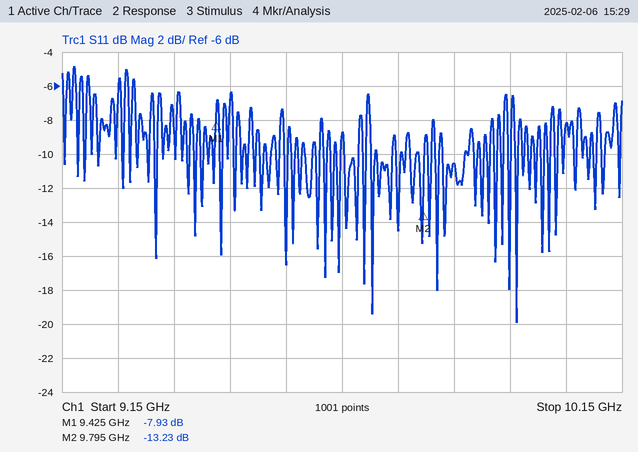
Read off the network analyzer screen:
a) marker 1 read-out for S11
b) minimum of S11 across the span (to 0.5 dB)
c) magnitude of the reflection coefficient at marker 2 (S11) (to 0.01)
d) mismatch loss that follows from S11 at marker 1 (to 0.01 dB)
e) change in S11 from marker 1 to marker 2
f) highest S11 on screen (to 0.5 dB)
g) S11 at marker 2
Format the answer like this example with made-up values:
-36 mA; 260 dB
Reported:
-7.93 dB; -20.0 dB; 0.22; 0.76 dB; -5.30 dB; -5.0 dB; -13.23 dB
